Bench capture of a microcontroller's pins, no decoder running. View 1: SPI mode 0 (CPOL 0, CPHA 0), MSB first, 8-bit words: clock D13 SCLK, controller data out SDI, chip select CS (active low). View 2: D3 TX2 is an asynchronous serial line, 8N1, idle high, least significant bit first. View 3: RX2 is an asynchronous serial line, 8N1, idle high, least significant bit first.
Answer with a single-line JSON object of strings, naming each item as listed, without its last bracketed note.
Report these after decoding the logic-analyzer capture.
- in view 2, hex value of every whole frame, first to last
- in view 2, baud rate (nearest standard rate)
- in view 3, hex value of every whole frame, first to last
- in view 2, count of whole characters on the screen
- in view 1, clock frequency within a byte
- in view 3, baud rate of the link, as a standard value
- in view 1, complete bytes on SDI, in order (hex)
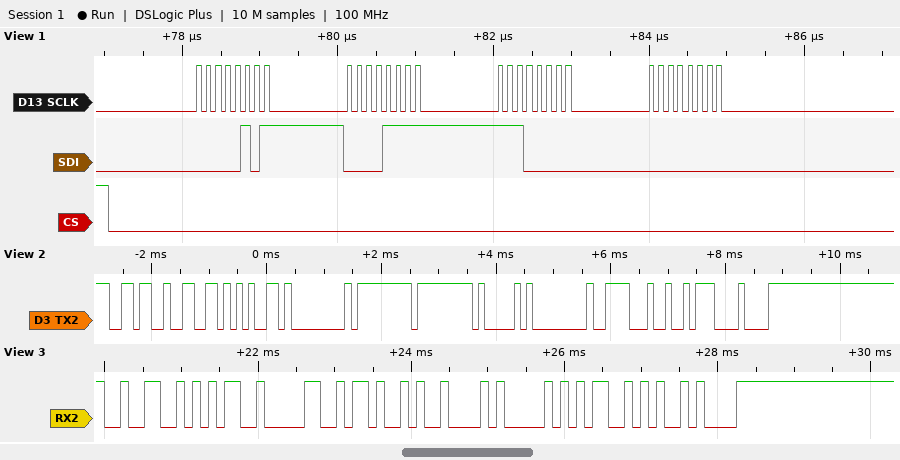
{"in view 2, hex value of every whole frame, first to last": "36 66 65 00 FF FF 41 00 1E D2 08", "in view 2, baud rate": "9600 baud", "in view 3, hex value of every whole frame, first to last": "32 35 30 4B 42 50 53 0A", "in view 2, count of whole characters on the screen": "11", "in view 1, clock frequency within a byte": "8 MHz", "in view 3, baud rate of the link, as a standard value": "9600 baud", "in view 1, complete bytes on SDI, in order": "05 0F E0 00"}
